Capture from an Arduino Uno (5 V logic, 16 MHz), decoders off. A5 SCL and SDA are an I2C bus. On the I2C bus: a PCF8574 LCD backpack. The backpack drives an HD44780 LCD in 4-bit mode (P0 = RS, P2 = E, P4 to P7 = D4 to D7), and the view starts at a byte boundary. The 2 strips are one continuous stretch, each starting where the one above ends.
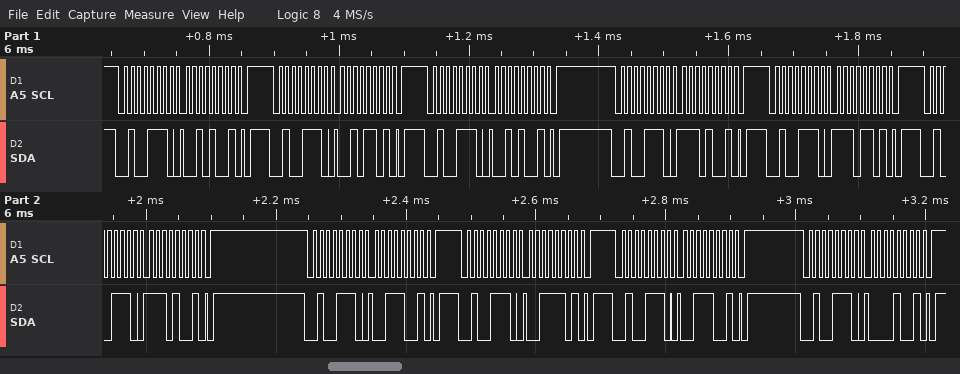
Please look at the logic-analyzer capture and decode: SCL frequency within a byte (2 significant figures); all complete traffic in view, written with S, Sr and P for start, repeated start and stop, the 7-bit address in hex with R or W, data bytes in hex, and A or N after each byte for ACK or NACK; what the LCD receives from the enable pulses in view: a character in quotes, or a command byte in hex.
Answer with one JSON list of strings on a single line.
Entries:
["100 kHz", "S 27W A 29 A P S 27W A 2D A P S 27W A 29 A P S 27W A E9 A P S 27W A ED A P S 27W A E9 A P S 27W A 39 A P S 27W A 3D A P S 27W A 39 A P S 27W A 09 A P", "'.'"]
